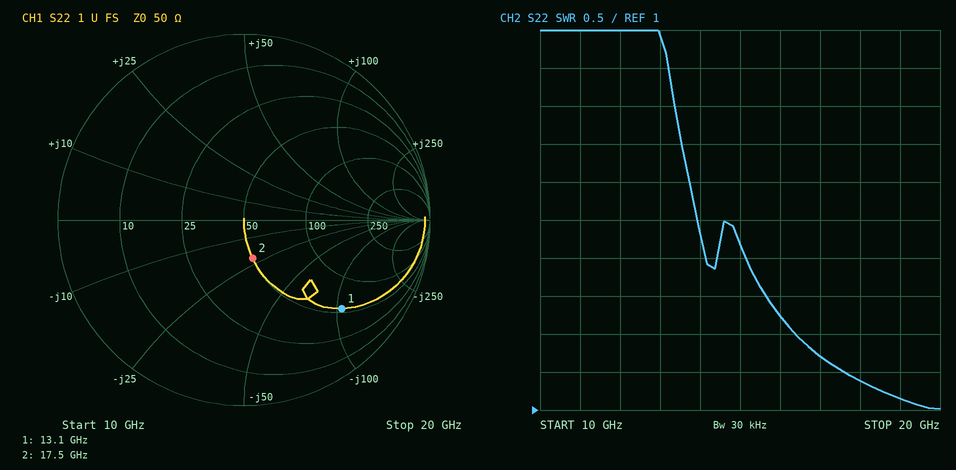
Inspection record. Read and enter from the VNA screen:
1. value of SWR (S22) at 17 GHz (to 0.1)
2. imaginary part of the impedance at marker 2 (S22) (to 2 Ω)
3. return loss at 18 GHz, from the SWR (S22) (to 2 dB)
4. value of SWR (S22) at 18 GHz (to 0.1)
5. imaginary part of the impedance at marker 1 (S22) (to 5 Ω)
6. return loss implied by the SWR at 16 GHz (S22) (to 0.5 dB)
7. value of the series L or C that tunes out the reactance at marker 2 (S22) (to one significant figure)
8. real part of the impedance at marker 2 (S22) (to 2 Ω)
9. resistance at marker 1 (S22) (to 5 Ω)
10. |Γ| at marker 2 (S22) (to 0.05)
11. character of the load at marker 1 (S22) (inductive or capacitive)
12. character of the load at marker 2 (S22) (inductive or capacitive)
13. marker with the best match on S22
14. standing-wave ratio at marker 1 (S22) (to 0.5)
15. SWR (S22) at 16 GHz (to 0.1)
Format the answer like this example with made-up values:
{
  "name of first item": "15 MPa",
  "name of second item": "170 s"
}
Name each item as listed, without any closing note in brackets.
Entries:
{
  "value of SWR (S22) at 17 GHz": "1.7",
  "imaginary part of the impedance at marker 2 (S22)": "-22 Ω",
  "return loss at 18 GHz, from the SWR (S22)": "16 dB",
  "value of SWR (S22) at 18 GHz": "1.4",
  "imaginary part of the impedance at marker 1 (S22)": "-105 Ω",
  "return loss implied by the SWR at 16 GHz (S22)": "8.5 dB",
  "value of the series L or C that tunes out the reactance at marker 2 (S22)": "200 pH",
  "real part of the impedance at marker 2 (S22)": "50 Ω",
  "resistance at marker 1 (S22)": "55 Ω",
  "|Γ| at marker 2 (S22)": "0.20",
  "character of the load at marker 1 (S22)": "capacitive",
  "character of the load at marker 2 (S22)": "capacitive",
  "marker with the best match on S22": "marker 2",
  "standing-wave ratio at marker 1 (S22)": "6.0",
  "SWR (S22) at 16 GHz": "2.2"
}
